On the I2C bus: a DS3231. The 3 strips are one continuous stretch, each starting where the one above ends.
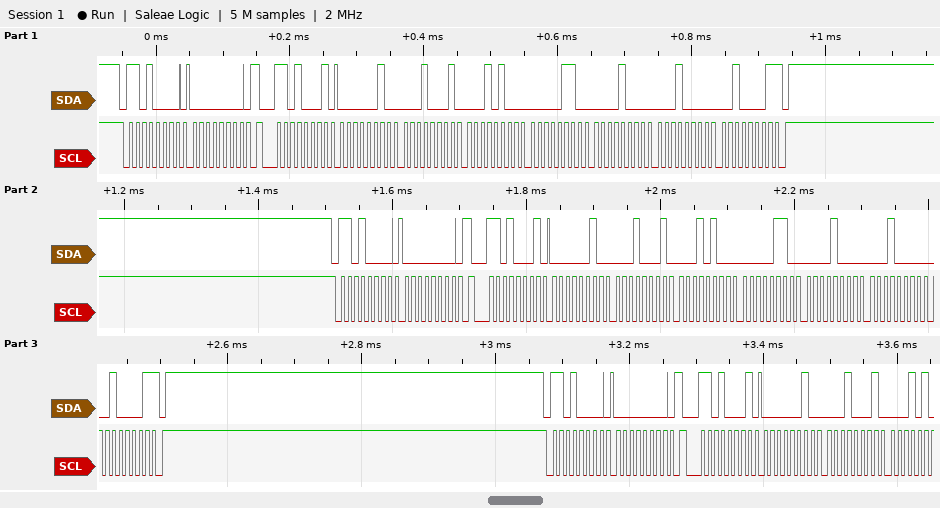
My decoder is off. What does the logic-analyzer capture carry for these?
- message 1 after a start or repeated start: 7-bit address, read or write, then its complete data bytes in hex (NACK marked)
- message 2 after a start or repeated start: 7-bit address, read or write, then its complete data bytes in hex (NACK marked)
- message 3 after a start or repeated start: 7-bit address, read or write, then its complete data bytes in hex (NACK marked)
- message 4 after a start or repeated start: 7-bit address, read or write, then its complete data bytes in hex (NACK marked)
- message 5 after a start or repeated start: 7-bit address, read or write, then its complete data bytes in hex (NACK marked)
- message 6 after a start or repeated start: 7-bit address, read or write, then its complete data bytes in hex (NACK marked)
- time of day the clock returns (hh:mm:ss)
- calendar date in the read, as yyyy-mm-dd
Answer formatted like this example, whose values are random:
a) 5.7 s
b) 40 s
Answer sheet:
a) 0x68 write: 00
b) 0x68 read: 02 11 14 06 08 10 21 NACK
c) 0x68 write: 00
d) 0x68 read: 02 11 14 06 08 10 21 NACK
e) 0x68 write: 00
f) 0x68 read: 02 11
g) 14:11:02
h) 2021-10-08
